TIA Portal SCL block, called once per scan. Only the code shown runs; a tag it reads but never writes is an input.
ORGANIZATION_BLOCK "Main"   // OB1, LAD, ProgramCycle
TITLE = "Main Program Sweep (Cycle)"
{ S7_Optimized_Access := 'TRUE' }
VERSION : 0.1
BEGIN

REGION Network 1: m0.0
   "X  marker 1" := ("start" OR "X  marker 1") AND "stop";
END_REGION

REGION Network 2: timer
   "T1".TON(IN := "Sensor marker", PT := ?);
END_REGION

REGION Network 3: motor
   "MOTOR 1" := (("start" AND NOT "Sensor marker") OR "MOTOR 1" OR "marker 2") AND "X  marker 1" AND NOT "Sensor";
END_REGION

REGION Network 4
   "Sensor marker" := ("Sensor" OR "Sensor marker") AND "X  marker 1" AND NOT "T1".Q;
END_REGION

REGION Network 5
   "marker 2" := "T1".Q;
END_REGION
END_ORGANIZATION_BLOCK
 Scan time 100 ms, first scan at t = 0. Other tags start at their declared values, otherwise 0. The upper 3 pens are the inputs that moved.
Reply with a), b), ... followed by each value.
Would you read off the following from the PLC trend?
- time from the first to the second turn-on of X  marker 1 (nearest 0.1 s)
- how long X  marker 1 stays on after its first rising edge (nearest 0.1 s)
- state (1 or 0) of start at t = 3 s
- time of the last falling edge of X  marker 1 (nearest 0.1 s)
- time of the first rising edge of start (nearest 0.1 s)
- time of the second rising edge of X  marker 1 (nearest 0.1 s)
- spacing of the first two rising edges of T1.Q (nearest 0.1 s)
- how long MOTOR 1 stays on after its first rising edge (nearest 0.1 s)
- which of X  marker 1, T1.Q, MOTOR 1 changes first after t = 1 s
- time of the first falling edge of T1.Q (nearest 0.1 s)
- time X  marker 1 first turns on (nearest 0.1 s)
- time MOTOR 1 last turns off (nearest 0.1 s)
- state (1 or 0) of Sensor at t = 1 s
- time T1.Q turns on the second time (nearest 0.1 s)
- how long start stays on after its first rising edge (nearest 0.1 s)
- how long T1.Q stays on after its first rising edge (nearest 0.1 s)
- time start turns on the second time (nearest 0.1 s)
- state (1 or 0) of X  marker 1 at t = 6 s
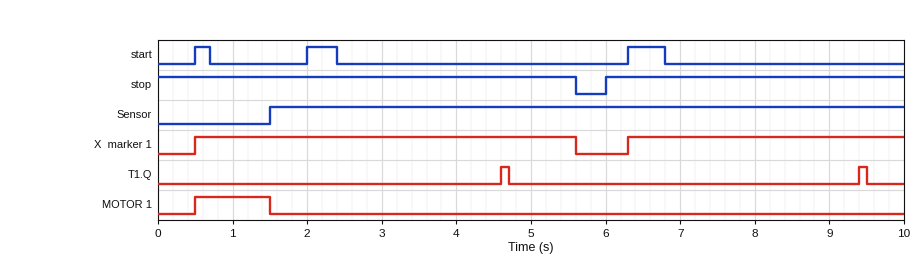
a) 5.8 s
b) 5.1 s
c) 0
d) 5.6 s
e) 0.5 s
f) 6.3 s
g) 4.8 s
h) 1.0 s
i) MOTOR 1
j) 4.7 s
k) 0.5 s
l) 1.5 s
m) 0
n) 9.4 s
o) 0.2 s
p) 0.1 s
q) 2.0 s
r) 0
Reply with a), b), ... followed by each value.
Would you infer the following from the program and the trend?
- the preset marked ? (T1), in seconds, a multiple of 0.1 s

a) 3.0 s
